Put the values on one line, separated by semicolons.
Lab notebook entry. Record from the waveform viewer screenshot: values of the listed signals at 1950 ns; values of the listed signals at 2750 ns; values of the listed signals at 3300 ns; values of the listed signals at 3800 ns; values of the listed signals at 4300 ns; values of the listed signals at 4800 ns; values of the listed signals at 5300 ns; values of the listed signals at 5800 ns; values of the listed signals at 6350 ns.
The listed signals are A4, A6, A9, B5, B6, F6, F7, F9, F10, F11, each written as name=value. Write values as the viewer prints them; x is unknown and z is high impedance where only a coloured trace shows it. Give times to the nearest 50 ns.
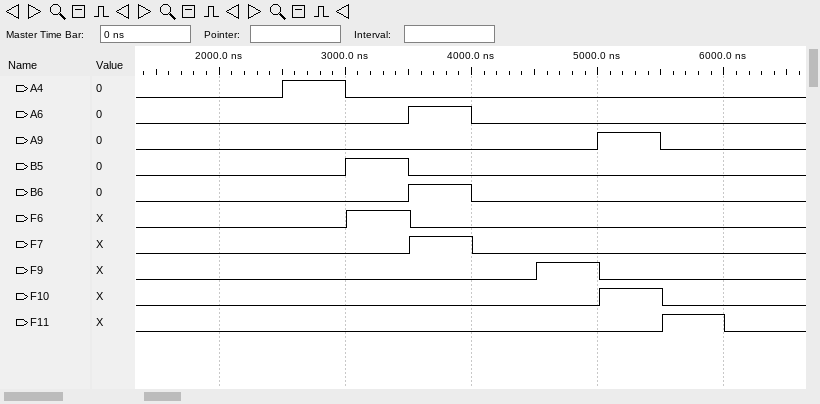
A4=0, A6=0, A9=0, B5=0, B6=0, F6=0, F7=0, F9=0, F10=0, F11=0; A4=1, A6=0, A9=0, B5=0, B6=0, F6=0, F7=0, F9=0, F10=0, F11=0; A4=0, A6=0, A9=0, B5=1, B6=0, F6=1, F7=0, F9=0, F10=0, F11=0; A4=0, A6=1, A9=0, B5=0, B6=1, F6=0, F7=1, F9=0, F10=0, F11=0; A4=0, A6=0, A9=0, B5=0, B6=0, F6=0, F7=0, F9=0, F10=0, F11=0; A4=0, A6=0, A9=0, B5=0, B6=0, F6=0, F7=0, F9=1, F10=0, F11=0; A4=0, A6=0, A9=1, B5=0, B6=0, F6=0, F7=0, F9=0, F10=1, F11=0; A4=0, A6=0, A9=0, B5=0, B6=0, F6=0, F7=0, F9=0, F10=0, F11=1; A4=0, A6=0, A9=0, B5=0, B6=0, F6=0, F7=0, F9=0, F10=0, F11=0
